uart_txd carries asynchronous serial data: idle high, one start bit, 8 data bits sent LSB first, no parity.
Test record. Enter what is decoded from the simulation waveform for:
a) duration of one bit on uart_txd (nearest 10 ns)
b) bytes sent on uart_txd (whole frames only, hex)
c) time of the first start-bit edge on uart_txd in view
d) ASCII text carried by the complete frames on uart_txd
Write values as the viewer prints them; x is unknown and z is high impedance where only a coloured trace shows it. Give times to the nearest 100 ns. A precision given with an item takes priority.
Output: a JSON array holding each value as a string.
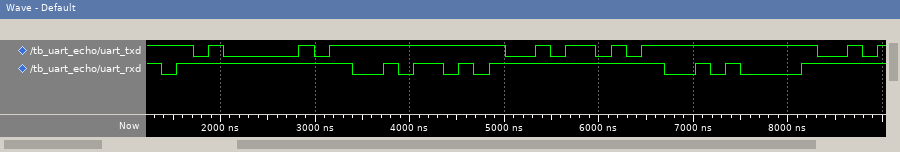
["160 ns", "41, 5A", "1700 ns", "\"AZ\""]
